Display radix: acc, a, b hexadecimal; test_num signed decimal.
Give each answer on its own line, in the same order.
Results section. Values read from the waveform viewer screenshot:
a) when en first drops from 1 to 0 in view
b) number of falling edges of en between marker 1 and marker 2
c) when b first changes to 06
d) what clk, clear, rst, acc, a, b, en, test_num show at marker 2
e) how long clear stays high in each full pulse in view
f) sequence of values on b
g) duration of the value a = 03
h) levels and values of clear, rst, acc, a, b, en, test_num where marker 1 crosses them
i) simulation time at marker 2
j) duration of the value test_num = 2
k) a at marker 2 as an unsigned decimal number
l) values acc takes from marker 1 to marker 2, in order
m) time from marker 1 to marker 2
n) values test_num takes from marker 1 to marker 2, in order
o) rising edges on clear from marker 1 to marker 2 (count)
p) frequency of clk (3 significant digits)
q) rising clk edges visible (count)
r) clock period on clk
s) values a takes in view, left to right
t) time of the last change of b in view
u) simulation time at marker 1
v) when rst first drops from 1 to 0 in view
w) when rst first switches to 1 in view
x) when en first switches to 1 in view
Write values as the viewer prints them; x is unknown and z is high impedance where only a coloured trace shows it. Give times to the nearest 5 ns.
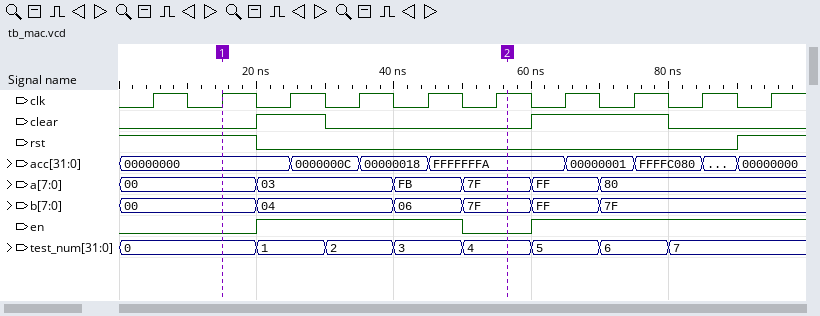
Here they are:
50 ns
1
40 ns
clk=1, clear=0, rst=0, acc=FFFFFFFA, a=7F, b=7F, en=0, test_num=4
10 ns, 20 ns
00, 04, 06, 7F, FF, 7F
20 ns
clear=0, rst=1, acc=00000000, a=00, b=00, en=0, test_num=0
55 ns
10 ns
127
00000000, 0000000C, 00000018, FFFFFFFA
40 ns
0, 1, 2, 3, 4
1
100 MHz
10
10 ns
00, 03, FB, 7F, FF, 80
70 ns
15 ns
20 ns
90 ns
20 ns
